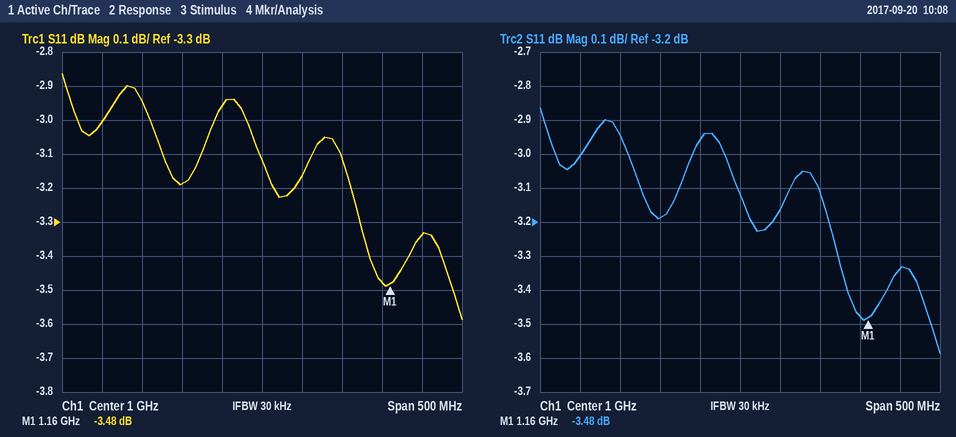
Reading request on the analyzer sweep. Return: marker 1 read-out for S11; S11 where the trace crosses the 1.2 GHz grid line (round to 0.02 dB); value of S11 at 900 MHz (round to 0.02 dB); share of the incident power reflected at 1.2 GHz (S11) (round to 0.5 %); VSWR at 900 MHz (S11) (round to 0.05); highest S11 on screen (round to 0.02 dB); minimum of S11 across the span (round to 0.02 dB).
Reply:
-3.48 dB
-3.34 dB
-3.18 dB
46.5 %
5.50
-2.86 dB
-3.58 dB
